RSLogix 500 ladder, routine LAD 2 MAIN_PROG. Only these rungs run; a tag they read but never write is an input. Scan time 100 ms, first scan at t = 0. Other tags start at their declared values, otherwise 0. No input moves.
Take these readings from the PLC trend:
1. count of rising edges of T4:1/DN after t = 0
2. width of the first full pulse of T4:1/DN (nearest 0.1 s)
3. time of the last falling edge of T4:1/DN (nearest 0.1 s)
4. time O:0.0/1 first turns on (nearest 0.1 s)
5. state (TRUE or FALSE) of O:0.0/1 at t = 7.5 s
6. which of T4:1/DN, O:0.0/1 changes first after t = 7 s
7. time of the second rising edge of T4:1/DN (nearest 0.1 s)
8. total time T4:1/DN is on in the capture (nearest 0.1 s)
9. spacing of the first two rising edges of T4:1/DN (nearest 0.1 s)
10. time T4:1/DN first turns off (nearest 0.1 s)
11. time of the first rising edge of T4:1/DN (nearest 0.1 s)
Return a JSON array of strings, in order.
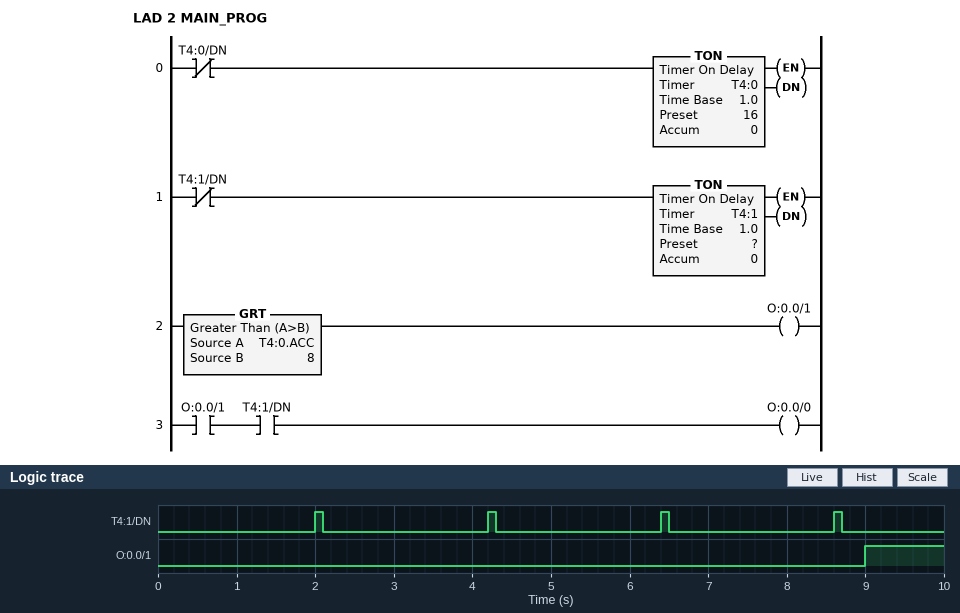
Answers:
["4", "0.1 s", "8.7 s", "9.0 s", "FALSE", "T4:1/DN", "4.2 s", "0.4 s", "2.2 s", "2.1 s", "2.0 s"]
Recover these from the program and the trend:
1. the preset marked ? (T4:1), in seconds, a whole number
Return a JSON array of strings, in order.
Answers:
["2 s"]
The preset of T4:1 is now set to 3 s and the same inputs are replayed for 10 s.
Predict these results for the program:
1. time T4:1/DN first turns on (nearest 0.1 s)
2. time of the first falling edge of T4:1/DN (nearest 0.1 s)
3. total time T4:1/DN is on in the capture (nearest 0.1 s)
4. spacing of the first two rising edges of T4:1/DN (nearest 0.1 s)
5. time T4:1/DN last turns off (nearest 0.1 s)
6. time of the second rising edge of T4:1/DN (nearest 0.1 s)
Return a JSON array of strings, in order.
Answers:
["3.0 s", "3.1 s", "0.3 s", "3.2 s", "9.5 s", "6.2 s"]
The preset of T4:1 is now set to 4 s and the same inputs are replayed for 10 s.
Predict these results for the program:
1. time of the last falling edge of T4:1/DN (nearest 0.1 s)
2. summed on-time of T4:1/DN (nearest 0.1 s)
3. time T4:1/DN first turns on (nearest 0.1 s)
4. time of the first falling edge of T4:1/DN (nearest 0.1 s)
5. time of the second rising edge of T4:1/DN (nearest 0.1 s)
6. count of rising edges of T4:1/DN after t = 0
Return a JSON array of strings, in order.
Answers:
["8.3 s", "0.2 s", "4.0 s", "4.1 s", "8.2 s", "2"]
